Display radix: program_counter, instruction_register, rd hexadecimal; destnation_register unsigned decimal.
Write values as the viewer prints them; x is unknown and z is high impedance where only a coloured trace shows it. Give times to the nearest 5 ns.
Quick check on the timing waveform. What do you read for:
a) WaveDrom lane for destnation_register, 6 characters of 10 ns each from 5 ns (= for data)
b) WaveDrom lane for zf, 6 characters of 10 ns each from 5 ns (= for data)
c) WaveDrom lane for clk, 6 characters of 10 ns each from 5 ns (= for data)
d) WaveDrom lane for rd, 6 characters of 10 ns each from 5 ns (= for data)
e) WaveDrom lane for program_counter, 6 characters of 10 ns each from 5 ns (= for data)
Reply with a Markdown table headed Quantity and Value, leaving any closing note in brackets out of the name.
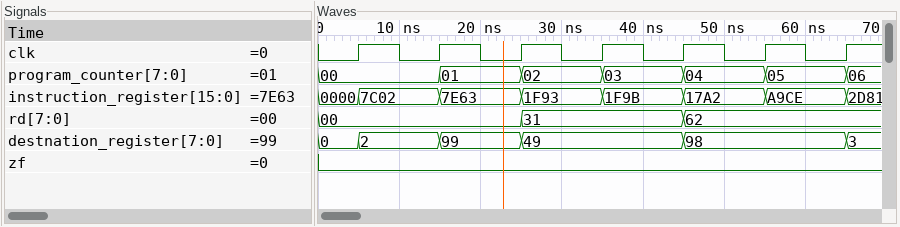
| Quantity | Value |
|---|---|
| WaveDrom lane for destnation_register, 6 characters of 10 ns each from 5 ns | {name: 'destnation_register', wave: '===.=.', data: '2 99 49 98'} |
| WaveDrom lane for zf, 6 characters of 10 ns each from 5 ns | {name: 'zf', wave: '0.....'} |
| WaveDrom lane for clk, 6 characters of 10 ns each from 5 ns | {name: 'clk', wave: 'p.....'} |
| WaveDrom lane for rd, 6 characters of 10 ns each from 5 ns | {name: 'rd', wave: '=.=.=.', data: '00 31 62'} |
| WaveDrom lane for program_counter, 6 characters of 10 ns each from 5 ns | {name: 'program_counter', wave: '======', data: '00 01 02 03 04 05'} |
